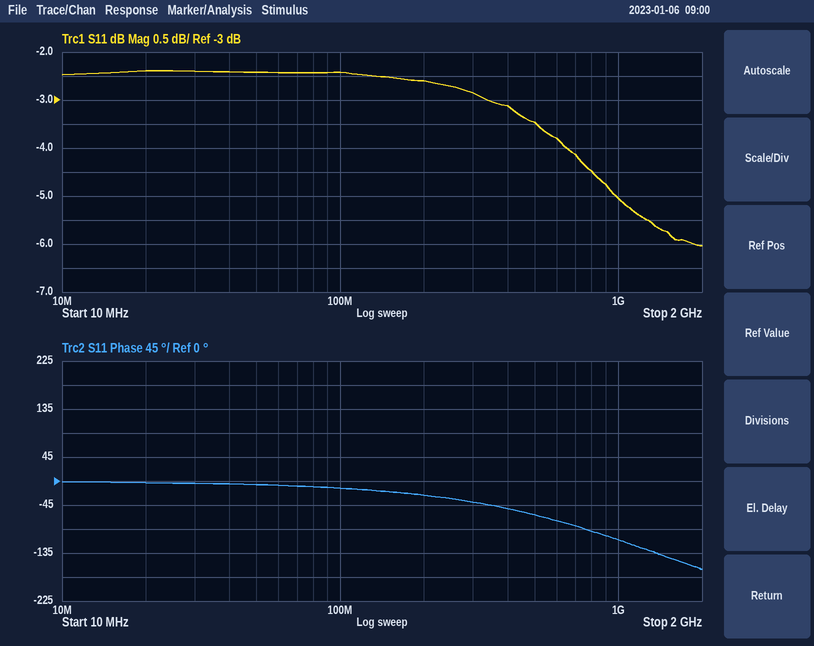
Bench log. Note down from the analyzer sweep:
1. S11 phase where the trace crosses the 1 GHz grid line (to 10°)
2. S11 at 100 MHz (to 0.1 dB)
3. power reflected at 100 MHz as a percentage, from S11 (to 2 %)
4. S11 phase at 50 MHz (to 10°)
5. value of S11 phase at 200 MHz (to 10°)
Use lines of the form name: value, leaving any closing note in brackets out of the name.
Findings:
S11 phase where the trace crosses the 1 GHz grid line: -110°
S11 at 100 MHz: -2.4 dB
power reflected at 100 MHz as a percentage, from S11: 58 %
S11 phase at 50 MHz: -10°
value of S11 phase at 200 MHz: -30°
